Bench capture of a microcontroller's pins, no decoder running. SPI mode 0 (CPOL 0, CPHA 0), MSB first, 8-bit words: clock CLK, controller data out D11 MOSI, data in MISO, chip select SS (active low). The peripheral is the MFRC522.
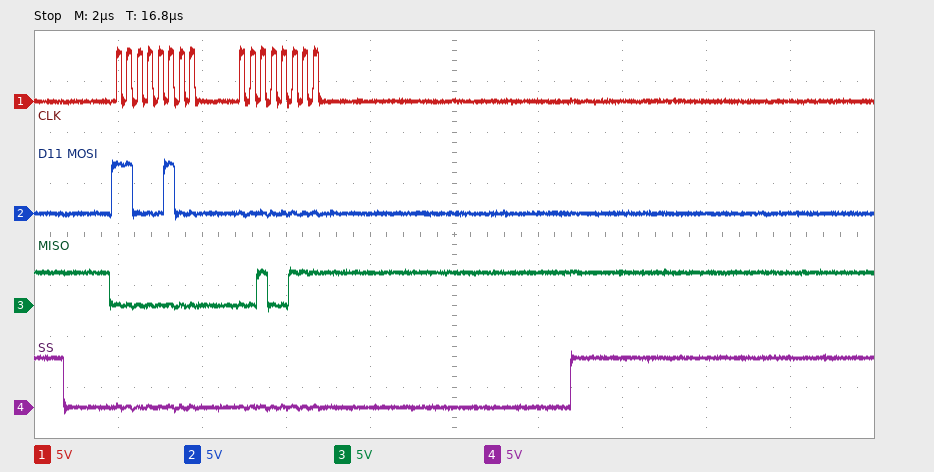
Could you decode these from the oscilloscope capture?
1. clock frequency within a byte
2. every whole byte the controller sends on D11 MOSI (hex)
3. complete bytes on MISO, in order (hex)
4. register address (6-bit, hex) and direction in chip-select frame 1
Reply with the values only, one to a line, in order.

4 MHz
0xC4 0x00
0x00 0x27
0x22 read
